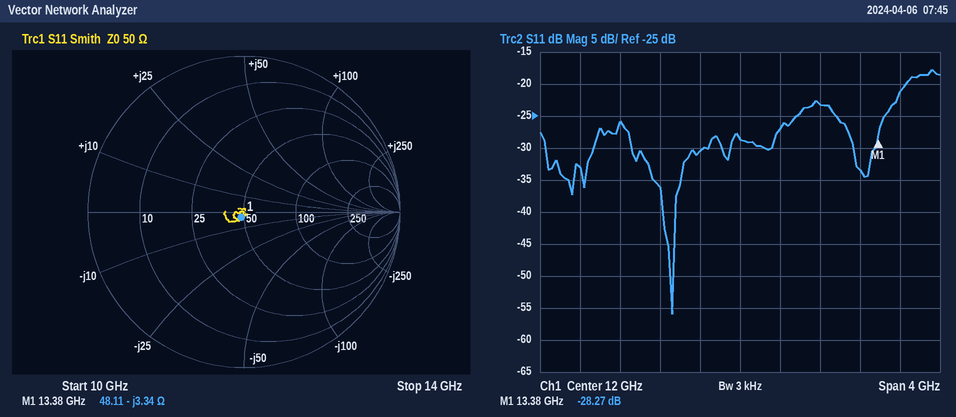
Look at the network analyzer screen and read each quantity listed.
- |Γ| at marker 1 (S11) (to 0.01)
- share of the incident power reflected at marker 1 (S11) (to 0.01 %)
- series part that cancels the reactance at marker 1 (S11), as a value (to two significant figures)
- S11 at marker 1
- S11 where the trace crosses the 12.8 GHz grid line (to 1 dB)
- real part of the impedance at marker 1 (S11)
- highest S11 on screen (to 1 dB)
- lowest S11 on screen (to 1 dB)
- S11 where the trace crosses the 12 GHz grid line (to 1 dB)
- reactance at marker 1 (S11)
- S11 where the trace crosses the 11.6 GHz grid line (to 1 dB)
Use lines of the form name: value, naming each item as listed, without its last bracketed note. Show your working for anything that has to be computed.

|Γ| at marker 1 (S11): 0.04
share of the incident power reflected at marker 1 (S11): 10^(-28.27/10) ≈ 0.15 %
series part that cancels the reactance at marker 1 (S11), as a value: L = 3.34 Ω/(2π × 13.38 GHz) ≈ 40 pH
S11 at marker 1: -28.27 dB
S11 where the trace crosses the 12.8 GHz grid line: -23 dB
real part of the impedance at marker 1: 48.11 Ω
highest S11 on screen: -18 dB
lowest S11 on screen: -56 dB
S11 where the trace crosses the 12 GHz grid line: -29 dB
reactance at marker 1: -3.34 Ω
S11 where the trace crosses the 11.6 GHz grid line: -30 dB
